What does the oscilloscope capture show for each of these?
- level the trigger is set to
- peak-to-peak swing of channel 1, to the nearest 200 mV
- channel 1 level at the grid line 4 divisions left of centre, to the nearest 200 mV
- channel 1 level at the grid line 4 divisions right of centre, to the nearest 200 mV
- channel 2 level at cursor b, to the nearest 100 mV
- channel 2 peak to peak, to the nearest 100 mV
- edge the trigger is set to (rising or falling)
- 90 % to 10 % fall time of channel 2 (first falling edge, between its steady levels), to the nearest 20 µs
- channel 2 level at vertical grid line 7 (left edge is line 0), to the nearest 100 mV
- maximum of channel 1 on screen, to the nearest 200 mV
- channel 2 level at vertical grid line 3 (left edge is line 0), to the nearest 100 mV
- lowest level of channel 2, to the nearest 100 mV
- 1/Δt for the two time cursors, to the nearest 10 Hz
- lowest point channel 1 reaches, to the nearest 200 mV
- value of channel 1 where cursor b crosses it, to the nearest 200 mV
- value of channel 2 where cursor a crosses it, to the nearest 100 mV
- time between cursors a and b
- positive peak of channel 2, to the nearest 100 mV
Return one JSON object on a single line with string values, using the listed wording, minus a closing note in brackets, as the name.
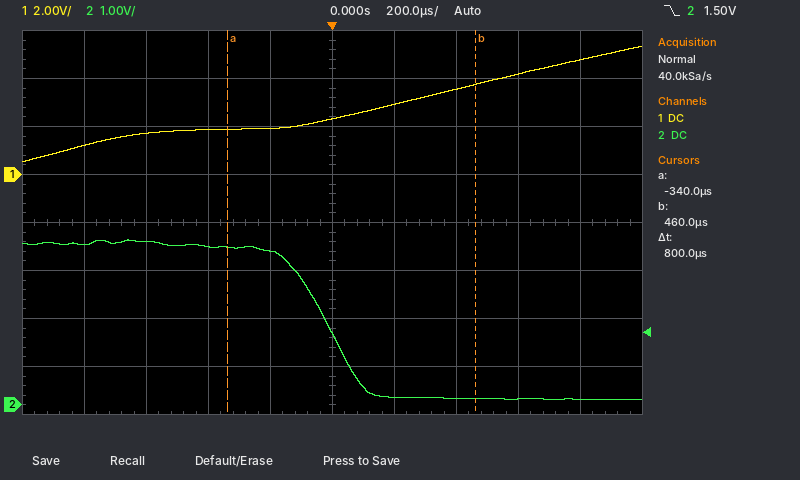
{"level the trigger is set to": "1.50 V", "peak-to-peak swing of channel 1, to the nearest 200 mV": "4.8 V", "channel 1 level at the grid line 4 divisions left of centre, to the nearest 200 mV": "1.2 V", "channel 1 level at the grid line 4 divisions right of centre, to the nearest 200 mV": "4.8 V", "channel 2 level at cursor b, to the nearest 100 mV": "100 mV", "channel 2 peak to peak, to the nearest 100 mV": "3.3 V", "edge the trigger is set to": "falling", "90 % to 10 % fall time of channel 2 (first falling edge, between its steady levels), to the nearest 20 µs": "240 µs", "channel 2 level at vertical grid line 7 (left edge is line 0), to the nearest 100 mV": "100 mV", "maximum of channel 1 on screen, to the nearest 200 mV": "5.4 V", "channel 2 level at vertical grid line 3 (left edge is line 0), to the nearest 100 mV": "3.3 V", "lowest level of channel 2, to the nearest 100 mV": "100 mV", "1/Δt for the two time cursors, to the nearest 10 Hz": "1.25 kHz", "lowest point channel 1 reaches, to the nearest 200 mV": "600 mV", "value of channel 1 where cursor b crosses it, to the nearest 200 mV": "3.8 V", "value of channel 2 where cursor a crosses it, to the nearest 100 mV": "3.3 V", "time between cursors a and b": "800 µs", "positive peak of channel 2, to the nearest 100 mV": "3.4 V"}
